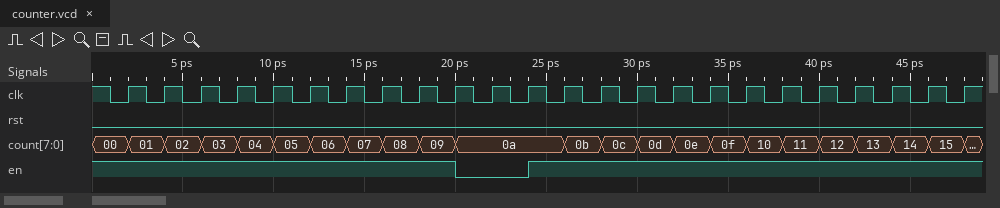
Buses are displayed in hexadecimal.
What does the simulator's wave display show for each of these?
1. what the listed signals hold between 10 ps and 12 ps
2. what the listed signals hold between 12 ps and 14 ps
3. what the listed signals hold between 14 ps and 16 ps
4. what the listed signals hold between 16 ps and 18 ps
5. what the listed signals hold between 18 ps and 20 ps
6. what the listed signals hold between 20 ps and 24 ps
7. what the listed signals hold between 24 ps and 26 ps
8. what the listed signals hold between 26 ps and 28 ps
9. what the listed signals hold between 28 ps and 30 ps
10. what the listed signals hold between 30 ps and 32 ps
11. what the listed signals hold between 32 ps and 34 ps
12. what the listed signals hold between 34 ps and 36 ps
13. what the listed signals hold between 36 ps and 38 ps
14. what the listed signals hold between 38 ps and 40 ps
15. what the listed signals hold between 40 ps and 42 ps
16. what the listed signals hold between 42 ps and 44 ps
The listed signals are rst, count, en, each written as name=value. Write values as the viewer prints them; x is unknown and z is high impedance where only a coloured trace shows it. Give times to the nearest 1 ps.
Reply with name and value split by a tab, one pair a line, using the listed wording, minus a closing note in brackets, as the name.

what the listed signals hold between 10 ps and 12 ps	rst=0, count=05, en=1
what the listed signals hold between 12 ps and 14 ps	rst=0, count=06, en=1
what the listed signals hold between 14 ps and 16 ps	rst=0, count=07, en=1
what the listed signals hold between 16 ps and 18 ps	rst=0, count=08, en=1
what the listed signals hold between 18 ps and 20 ps	rst=0, count=09, en=1
what the listed signals hold between 20 ps and 24 ps	rst=0, count=0a, en=0
what the listed signals hold between 24 ps and 26 ps	rst=0, count=0a, en=1
what the listed signals hold between 26 ps and 28 ps	rst=0, count=0b, en=1
what the listed signals hold between 28 ps and 30 ps	rst=0, count=0c, en=1
what the listed signals hold between 30 ps and 32 ps	rst=0, count=0d, en=1
what the listed signals hold between 32 ps and 34 ps	rst=0, count=0e, en=1
what the listed signals hold between 34 ps and 36 ps	rst=0, count=0f, en=1
what the listed signals hold between 36 ps and 38 ps	rst=0, count=10, en=1
what the listed signals hold between 38 ps and 40 ps	rst=0, count=11, en=1
what the listed signals hold between 40 ps and 42 ps	rst=0, count=12, en=1
what the listed signals hold between 42 ps and 44 ps	rst=0, count=13, en=1
